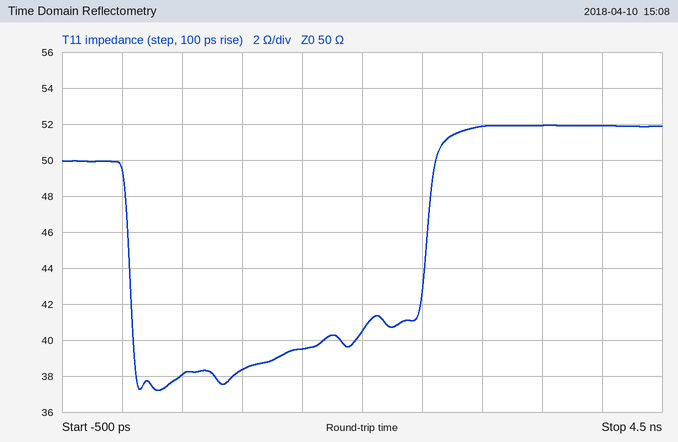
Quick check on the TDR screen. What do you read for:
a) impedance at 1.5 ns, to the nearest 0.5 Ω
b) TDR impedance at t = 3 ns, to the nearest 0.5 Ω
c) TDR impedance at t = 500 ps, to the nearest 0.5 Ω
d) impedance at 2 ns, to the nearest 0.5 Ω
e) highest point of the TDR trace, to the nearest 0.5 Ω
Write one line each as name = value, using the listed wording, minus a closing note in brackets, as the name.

impedance at 1.5 ns, to the nearest 0.5 Ω = 39.5 Ω
TDR impedance at t = 3 ns, to the nearest 0.5 Ω = 52.0 Ω
TDR impedance at t = 500 ps, to the nearest 0.5 Ω = 38.0 Ω
impedance at 2 ns, to the nearest 0.5 Ω = 40.5 Ω
highest point of the TDR trace, to the nearest 0.5 Ω = 52.0 Ω
